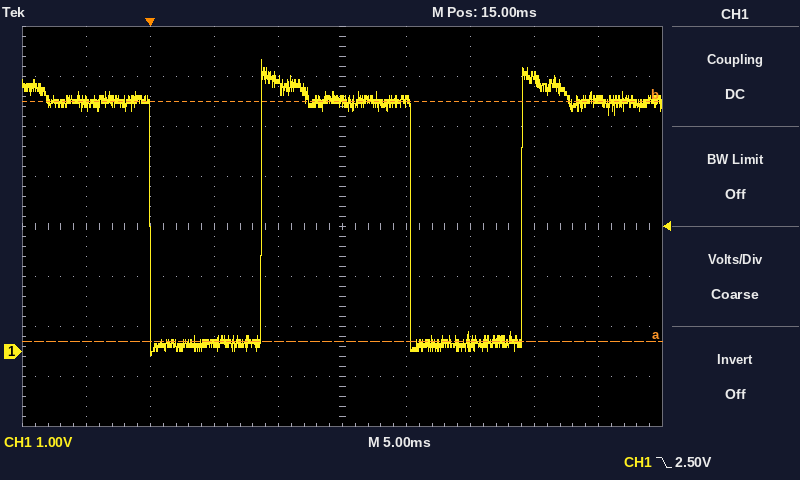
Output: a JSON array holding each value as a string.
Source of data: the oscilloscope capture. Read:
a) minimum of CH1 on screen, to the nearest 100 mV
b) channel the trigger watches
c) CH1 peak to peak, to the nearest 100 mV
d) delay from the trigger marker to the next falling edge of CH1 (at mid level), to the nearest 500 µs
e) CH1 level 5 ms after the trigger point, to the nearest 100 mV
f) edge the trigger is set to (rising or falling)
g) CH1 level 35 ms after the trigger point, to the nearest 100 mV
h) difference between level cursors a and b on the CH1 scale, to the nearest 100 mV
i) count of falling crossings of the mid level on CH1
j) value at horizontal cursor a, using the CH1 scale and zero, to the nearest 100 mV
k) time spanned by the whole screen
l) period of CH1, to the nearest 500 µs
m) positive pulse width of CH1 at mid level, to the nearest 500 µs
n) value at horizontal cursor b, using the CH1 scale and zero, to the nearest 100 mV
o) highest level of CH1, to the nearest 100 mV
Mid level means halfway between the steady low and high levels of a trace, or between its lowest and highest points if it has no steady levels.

["-100 mV", "CH1", "5.9 V", "20.5 ms", "200 mV", "falling", "5.0 V", "4.8 V", "2", "200 mV", "50 ms", "20.5 ms", "11.5 ms", "5.0 V", "5.8 V"]
